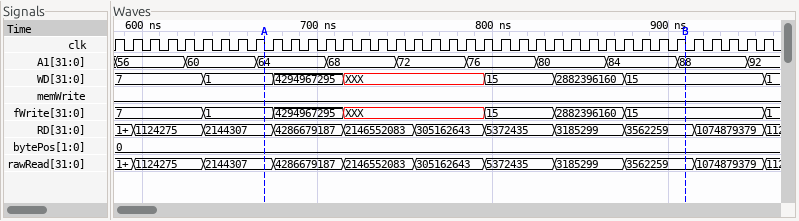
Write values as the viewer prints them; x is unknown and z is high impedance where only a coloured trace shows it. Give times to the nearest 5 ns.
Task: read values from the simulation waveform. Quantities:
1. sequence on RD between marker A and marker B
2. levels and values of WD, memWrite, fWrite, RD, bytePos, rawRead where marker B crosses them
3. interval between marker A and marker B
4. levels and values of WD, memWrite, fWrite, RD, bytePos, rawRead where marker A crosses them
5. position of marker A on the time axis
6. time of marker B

2144307, 4286679187, 2146552083, 305162643, 5372435, 3185299, 3562259
WD=15, memWrite=0, fWrite=15, RD=3562259, bytePos=0, rawRead=3562259
240 ns
WD=1, memWrite=0, fWrite=1, RD=2144307, bytePos=0, rawRead=2144307
670 ns
910 ns
